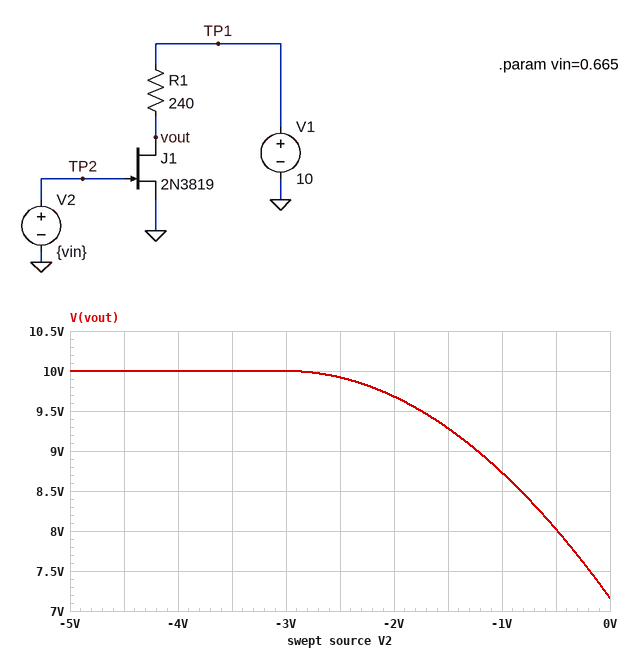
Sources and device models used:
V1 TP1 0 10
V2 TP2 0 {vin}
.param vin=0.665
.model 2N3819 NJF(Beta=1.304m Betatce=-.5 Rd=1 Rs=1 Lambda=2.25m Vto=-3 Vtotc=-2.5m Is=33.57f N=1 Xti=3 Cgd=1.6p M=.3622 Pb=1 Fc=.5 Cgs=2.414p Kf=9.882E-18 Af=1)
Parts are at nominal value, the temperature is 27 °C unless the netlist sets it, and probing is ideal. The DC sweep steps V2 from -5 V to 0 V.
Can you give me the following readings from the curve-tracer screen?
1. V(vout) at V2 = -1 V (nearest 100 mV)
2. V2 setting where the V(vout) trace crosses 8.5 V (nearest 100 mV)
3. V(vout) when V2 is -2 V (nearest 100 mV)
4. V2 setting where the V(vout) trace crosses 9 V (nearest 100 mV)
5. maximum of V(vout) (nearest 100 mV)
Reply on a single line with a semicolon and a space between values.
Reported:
8.7 V; -800 mV; 9.7 V; -1.2 V; 10.0 V
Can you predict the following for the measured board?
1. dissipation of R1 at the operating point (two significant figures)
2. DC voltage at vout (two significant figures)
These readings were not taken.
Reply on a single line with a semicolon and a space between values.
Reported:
74 mW; 5.8 V
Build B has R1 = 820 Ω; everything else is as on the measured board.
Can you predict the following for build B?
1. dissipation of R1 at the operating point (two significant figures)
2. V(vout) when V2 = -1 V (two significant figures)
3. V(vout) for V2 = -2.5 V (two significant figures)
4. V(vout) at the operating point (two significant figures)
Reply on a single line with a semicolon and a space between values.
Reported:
91 mW; 5.7 V; 9.7 V; 1.4 V
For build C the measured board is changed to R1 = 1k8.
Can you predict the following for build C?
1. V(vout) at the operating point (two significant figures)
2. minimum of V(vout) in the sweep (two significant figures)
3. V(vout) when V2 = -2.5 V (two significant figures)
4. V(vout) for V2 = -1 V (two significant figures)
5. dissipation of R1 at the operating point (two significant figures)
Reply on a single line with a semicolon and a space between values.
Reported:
610 mV; 760 mV; 9.4 V; 1.4 V; 49 mW
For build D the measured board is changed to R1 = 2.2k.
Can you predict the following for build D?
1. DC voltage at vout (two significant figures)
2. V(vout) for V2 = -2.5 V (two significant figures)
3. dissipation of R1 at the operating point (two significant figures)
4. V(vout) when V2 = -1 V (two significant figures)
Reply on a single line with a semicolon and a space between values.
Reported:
500 mV; 9.3 V; 41 mW; 1.1 V
